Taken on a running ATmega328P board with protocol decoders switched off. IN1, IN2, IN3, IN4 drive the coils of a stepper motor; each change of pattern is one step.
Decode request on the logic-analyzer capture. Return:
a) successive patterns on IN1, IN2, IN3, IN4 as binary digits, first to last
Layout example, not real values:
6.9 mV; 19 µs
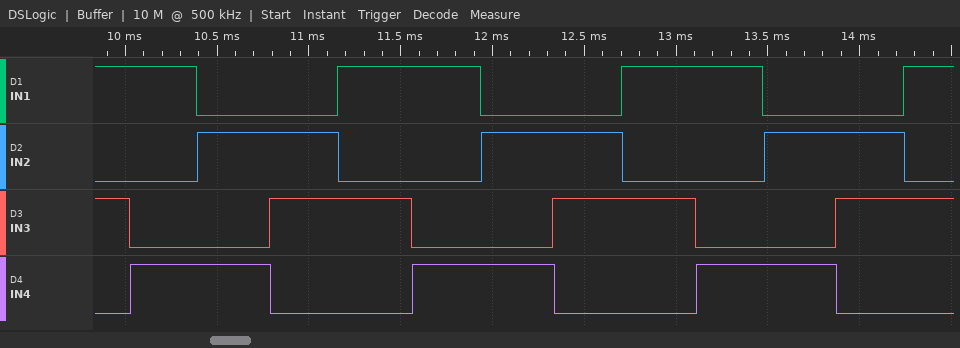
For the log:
1010 1001 0101 0110 1010 1001 0101 0110 1010 1001 0101 0110 1010
